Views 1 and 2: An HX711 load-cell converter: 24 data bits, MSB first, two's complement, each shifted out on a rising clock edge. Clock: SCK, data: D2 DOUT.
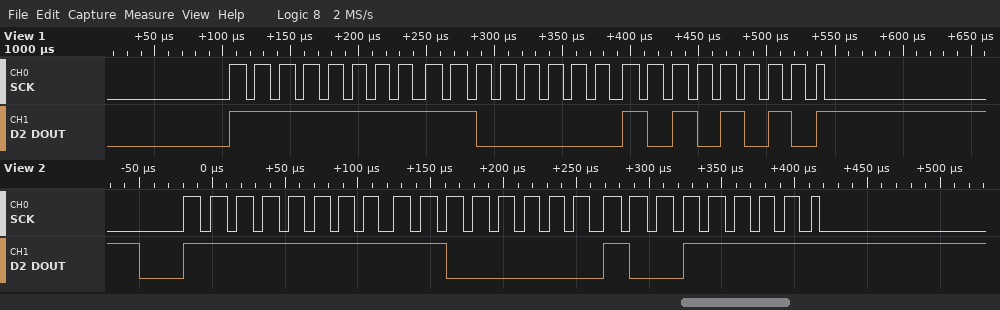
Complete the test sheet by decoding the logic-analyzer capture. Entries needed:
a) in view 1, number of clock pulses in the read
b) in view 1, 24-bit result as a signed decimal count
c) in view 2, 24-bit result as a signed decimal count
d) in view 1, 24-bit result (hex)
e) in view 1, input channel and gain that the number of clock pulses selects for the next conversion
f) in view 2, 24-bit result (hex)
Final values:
25
-16214
-16225
0xFFC0AA
channel A, gain 128
0xFFC09F
